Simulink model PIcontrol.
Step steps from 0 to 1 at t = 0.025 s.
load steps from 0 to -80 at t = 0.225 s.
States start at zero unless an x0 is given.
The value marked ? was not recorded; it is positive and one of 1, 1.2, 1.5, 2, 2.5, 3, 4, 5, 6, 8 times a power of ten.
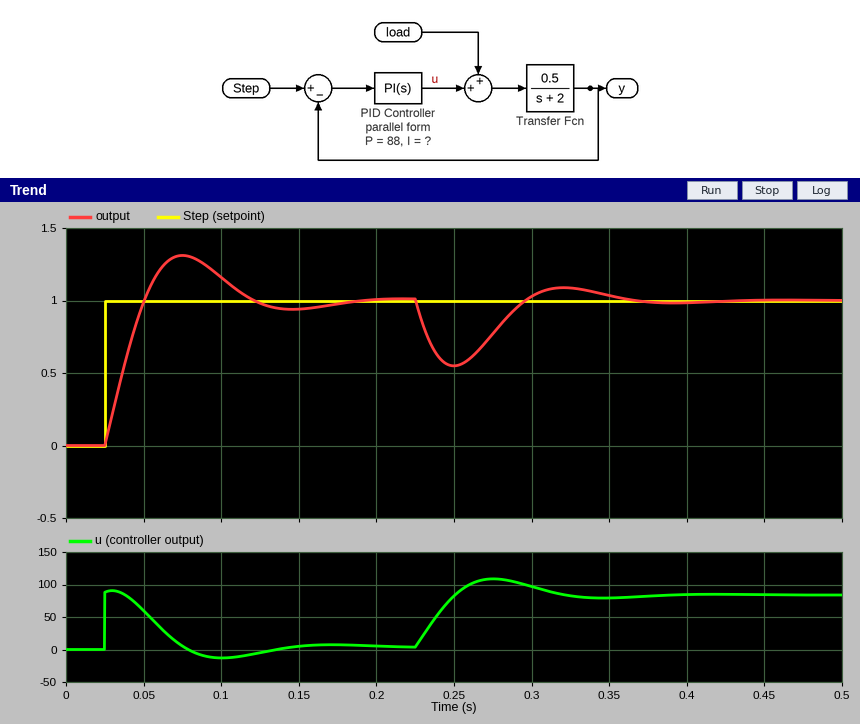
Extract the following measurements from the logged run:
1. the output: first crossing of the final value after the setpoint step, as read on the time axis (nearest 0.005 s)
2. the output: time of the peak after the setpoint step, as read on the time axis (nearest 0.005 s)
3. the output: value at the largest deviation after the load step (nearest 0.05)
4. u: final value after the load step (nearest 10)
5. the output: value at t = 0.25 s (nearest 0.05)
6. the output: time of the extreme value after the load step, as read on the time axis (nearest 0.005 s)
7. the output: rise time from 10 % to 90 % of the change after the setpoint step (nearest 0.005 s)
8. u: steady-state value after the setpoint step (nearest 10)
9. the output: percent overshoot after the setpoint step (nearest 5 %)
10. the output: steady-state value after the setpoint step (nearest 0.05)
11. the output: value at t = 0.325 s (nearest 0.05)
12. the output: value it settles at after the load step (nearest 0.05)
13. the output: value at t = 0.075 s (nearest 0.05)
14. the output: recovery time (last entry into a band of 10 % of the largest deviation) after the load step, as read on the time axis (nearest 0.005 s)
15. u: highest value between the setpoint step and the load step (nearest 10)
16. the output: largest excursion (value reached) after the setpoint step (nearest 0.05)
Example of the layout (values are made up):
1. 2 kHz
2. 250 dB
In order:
1. 0.050 s
2. 0.075 s
3. 0.55
4. 80
5. 0.55
6. 0.250 s
7. 0.020 s
8. 0
9. 30 %
10. 1.00
11. 1.10
12. 1.00
13. 1.30
14. 0.345 s
15. 90
16. 1.30
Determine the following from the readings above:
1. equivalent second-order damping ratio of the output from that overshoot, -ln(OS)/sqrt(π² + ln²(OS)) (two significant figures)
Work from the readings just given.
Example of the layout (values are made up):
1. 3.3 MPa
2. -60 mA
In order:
1. 0.36
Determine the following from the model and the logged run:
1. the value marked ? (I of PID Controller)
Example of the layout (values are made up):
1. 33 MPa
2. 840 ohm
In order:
1. 5000
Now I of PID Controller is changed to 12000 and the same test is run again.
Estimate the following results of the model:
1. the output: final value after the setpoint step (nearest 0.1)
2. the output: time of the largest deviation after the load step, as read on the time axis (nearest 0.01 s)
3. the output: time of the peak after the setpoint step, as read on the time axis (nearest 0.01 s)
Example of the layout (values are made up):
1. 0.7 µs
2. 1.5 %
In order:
1. 1.0
2. 0.24 s
3. 0.06 s
